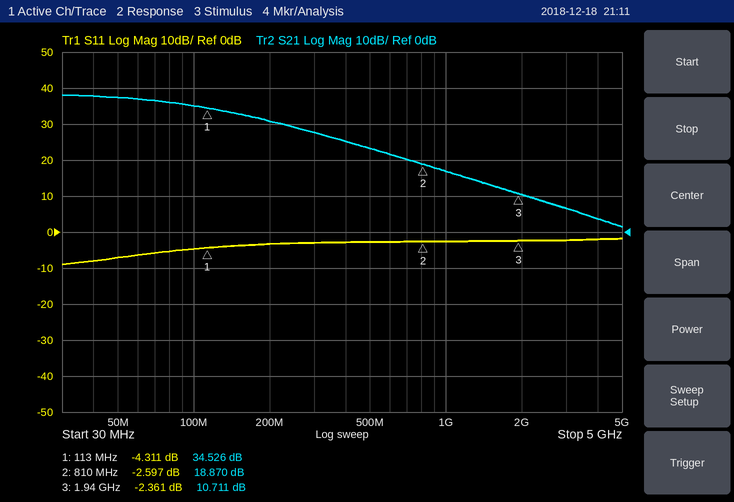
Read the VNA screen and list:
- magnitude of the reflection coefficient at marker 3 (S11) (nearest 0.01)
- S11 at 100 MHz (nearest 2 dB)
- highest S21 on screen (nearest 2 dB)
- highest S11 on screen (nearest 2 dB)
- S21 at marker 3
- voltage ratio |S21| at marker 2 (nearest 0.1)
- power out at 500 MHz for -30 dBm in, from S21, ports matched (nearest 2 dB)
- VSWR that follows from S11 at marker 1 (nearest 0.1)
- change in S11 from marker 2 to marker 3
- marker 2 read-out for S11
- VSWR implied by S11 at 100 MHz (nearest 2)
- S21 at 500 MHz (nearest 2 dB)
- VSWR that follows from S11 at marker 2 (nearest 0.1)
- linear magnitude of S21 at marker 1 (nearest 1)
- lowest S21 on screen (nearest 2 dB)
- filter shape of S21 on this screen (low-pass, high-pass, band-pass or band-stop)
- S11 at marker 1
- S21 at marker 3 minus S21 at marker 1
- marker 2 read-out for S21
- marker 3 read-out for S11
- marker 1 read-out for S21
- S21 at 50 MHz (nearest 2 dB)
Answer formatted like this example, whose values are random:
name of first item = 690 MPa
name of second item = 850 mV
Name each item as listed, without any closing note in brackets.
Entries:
magnitude of the reflection coefficient at marker 3 (S11) = 0.76
S11 at 100 MHz = -4 dB
highest S21 on screen = 38 dB
highest S11 on screen = -2 dB
S21 at marker 3 = 10.711 dB
voltage ratio |S21| at marker 2 = 8.8
power out at 500 MHz for -30 dBm in, from S21, ports matched = -6 dBm
VSWR that follows from S11 at marker 1 = 4.1
change in S11 from marker 2 to marker 3 = 0.236 dB
marker 2 read-out for S11 = -2.597 dB
VSWR implied by S11 at 100 MHz = 4
S21 at 500 MHz = 24 dB
VSWR that follows from S11 at marker 2 = 6.7
linear magnitude of S21 at marker 1 = 53
lowest S21 on screen = 2 dB
filter shape of S21 on this screen = low-pass
S11 at marker 1 = -4.311 dB
S21 at marker 3 minus S21 at marker 1 = -23.815 dB
marker 2 read-out for S21 = 18.870 dB
marker 3 read-out for S11 = -2.361 dB
marker 1 read-out for S21 = 34.526 dB
S21 at 50 MHz = 38 dB
